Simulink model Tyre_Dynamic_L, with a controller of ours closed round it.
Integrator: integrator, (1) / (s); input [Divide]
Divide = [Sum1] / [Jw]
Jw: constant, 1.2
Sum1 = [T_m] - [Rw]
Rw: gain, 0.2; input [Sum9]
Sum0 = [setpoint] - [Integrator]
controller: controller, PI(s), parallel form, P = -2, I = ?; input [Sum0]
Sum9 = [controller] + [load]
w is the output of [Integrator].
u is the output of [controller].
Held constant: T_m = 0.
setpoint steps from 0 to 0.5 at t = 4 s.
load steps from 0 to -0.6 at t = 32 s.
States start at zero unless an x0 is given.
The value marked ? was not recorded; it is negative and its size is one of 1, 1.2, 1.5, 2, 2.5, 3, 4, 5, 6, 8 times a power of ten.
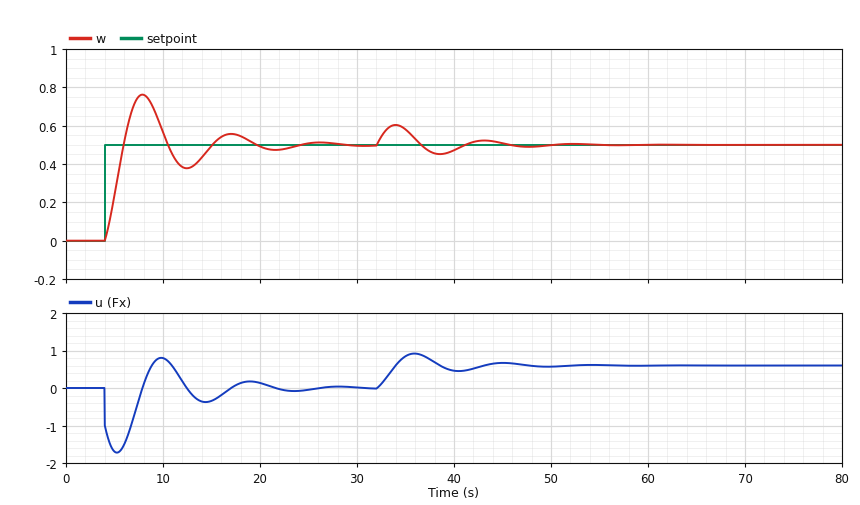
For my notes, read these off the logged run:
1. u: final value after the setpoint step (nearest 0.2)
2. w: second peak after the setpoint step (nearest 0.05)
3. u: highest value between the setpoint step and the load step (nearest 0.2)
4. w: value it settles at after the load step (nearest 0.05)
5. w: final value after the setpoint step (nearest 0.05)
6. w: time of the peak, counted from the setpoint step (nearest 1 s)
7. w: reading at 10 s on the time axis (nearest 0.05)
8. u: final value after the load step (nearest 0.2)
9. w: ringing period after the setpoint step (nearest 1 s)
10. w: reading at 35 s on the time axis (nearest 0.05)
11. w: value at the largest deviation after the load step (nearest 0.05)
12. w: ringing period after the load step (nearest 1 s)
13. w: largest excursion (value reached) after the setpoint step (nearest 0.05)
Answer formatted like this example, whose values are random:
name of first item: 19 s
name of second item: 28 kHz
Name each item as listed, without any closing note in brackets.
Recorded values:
u: final value after the setpoint step: 0.0
w: second peak after the setpoint step: 0.55
u: highest value between the setpoint step and the load step: 0.8
w: value it settles at after the load step: 0.50
w: final value after the setpoint step: 0.50
w: time of the peak, counted from the setpoint step: 4 s
w: reading at 10 s on the time axis: 0.55
u: final value after the load step: 0.6
w: ringing period after the setpoint step: 9 s
w: reading at 35 s on the time axis: 0.60
w: value at the largest deviation after the load step: 0.60
w: ringing period after the load step: 9 s
w: largest excursion (value reached) after the setpoint step: 0.75
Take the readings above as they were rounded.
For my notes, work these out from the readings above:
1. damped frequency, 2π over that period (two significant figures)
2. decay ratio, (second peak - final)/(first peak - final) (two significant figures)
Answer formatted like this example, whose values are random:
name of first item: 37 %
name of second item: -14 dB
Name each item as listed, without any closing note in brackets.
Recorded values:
damped frequency, 2π over that period: 0.70 rad/s
decay ratio, (second peak - final)/(first peak - final): 0.20
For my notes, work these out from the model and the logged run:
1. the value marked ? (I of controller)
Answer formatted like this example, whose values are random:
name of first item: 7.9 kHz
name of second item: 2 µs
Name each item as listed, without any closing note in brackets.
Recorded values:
the value marked ?: -3
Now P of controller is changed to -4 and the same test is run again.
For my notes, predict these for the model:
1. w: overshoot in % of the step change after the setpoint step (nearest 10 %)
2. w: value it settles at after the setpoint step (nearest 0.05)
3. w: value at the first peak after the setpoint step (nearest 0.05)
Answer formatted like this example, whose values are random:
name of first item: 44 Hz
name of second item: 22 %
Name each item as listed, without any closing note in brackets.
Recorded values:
w: overshoot in % of the step change after the setpoint step: 30 %
w: value it settles at after the setpoint step: 0.50
w: value at the first peak after the setpoint step: 0.65
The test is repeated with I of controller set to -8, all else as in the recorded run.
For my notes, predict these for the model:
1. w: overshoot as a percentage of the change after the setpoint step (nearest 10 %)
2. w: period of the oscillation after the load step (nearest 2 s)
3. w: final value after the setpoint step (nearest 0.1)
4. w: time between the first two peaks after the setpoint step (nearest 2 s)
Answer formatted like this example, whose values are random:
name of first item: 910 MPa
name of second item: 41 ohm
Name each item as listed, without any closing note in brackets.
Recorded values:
w: overshoot as a percentage of the change after the setpoint step: 70 %
w: period of the oscillation after the load step: 6 s
w: final value after the setpoint step: 0.5
w: time between the first two peaks after the setpoint step: 6 s
